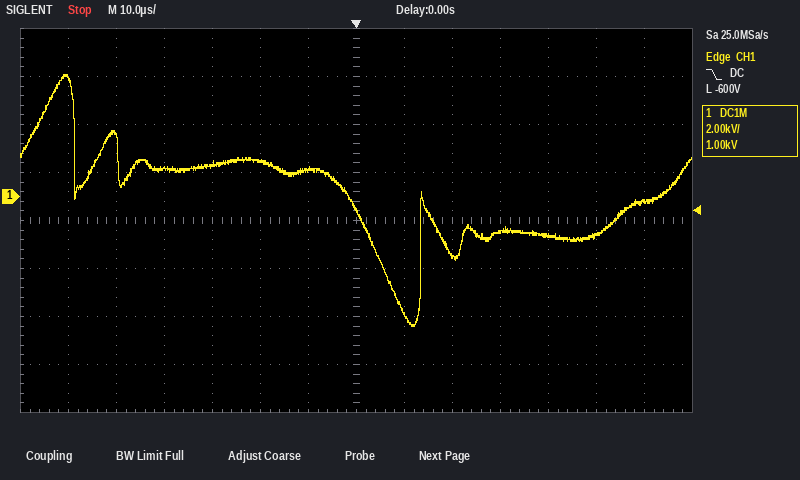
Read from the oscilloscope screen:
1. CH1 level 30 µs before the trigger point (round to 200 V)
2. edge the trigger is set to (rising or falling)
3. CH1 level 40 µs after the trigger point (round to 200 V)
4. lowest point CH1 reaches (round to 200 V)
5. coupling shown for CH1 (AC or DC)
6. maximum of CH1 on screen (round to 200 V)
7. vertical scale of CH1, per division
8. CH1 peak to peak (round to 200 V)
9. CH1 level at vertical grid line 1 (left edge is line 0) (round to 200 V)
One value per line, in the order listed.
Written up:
1.4 kV
falling
-1.6 kV
-5.4 kV
DC
5.0 kV
2 kV
10.4 kV
5.0 kV
